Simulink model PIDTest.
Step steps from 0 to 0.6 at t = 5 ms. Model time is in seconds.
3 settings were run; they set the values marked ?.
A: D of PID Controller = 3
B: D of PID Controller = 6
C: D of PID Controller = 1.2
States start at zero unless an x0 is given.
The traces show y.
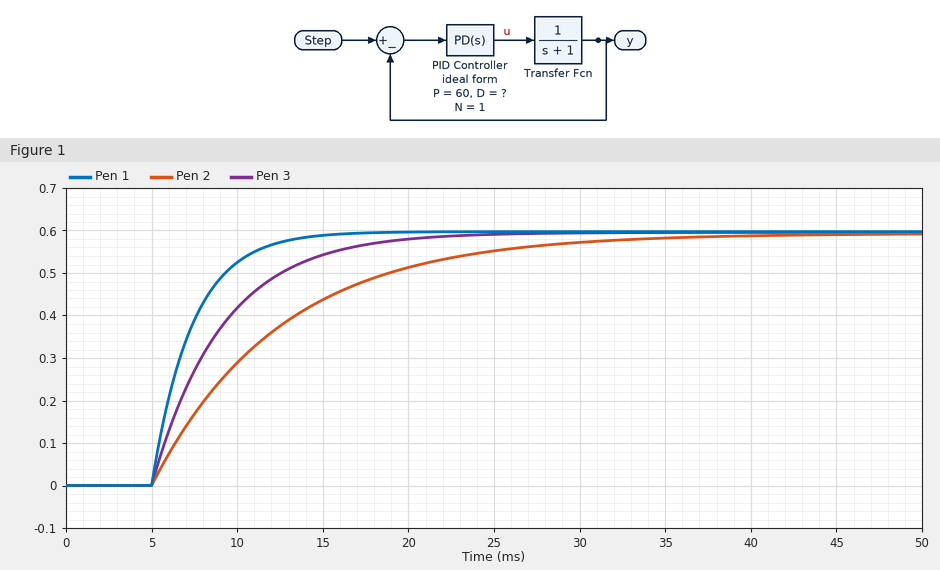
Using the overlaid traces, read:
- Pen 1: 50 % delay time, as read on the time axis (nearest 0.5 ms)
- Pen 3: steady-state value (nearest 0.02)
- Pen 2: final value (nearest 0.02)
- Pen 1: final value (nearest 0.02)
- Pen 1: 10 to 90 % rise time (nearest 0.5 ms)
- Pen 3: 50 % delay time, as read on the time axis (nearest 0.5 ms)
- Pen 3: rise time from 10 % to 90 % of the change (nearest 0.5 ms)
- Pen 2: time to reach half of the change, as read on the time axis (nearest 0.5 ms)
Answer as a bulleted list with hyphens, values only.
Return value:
- 6.5 ms
- 0.60
- 0.60
- 0.60
- 5.0 ms
- 8.0 ms
- 9.0 ms
- 10.0 ms
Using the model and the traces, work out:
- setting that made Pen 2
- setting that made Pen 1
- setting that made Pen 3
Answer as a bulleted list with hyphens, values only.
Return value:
- C
- B
- A
